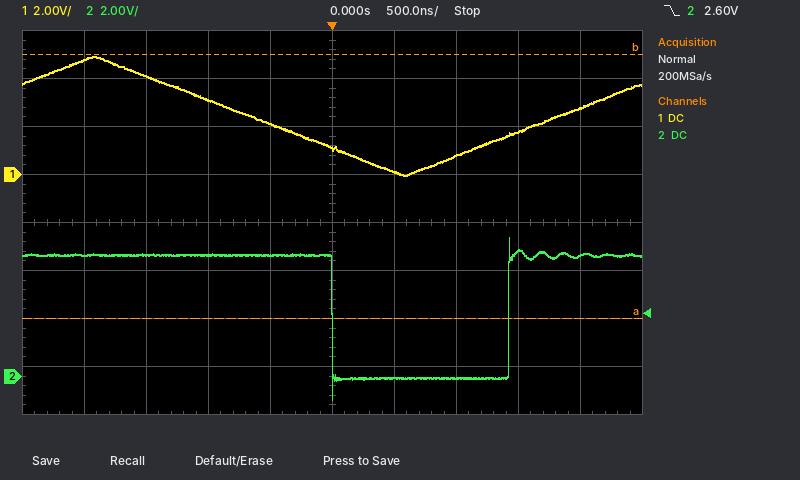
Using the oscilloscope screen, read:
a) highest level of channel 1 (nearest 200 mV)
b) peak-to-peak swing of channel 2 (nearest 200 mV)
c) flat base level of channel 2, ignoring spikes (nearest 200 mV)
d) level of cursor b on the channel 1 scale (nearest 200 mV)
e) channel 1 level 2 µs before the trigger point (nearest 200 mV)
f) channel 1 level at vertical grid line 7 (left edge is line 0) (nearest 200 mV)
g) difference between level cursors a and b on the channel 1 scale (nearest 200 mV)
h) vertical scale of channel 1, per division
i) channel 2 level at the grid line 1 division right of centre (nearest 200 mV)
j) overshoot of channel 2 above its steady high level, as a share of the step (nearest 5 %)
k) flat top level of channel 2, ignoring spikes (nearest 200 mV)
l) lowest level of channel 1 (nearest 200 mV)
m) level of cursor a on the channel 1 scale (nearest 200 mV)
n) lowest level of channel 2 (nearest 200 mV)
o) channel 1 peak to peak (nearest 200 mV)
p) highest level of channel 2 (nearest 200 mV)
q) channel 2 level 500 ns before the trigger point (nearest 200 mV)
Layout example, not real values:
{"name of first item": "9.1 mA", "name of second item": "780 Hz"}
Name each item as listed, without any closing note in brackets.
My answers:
{"highest level of channel 1": "5.0 V", "peak-to-peak swing of channel 2": "6.8 V", "flat base level of channel 2, ignoring spikes": "0.0 V", "level of cursor b on the channel 1 scale": "5.0 V", "channel 1 level 2 µs before the trigger point": "4.8 V", "channel 1 level at vertical grid line 7 (left edge is line 0)": "800 mV", "difference between level cursors a and b on the channel 1 scale": "11.0 V", "vertical scale of channel 1, per division": "2 V", "channel 2 level at the grid line 1 division right of centre": "0.0 V", "overshoot of channel 2 above its steady high level, as a share of the step": "15 %", "flat top level of channel 2, ignoring spikes": "5.0 V", "lowest level of channel 1": "0.0 V", "level of cursor a on the channel 1 scale": "-6.0 V", "lowest level of channel 2": "-1.0 V", "channel 1 peak to peak": "5.0 V", "highest level of channel 2": "5.8 V", "channel 2 level 500 ns before the trigger point": "5.0 V"}
